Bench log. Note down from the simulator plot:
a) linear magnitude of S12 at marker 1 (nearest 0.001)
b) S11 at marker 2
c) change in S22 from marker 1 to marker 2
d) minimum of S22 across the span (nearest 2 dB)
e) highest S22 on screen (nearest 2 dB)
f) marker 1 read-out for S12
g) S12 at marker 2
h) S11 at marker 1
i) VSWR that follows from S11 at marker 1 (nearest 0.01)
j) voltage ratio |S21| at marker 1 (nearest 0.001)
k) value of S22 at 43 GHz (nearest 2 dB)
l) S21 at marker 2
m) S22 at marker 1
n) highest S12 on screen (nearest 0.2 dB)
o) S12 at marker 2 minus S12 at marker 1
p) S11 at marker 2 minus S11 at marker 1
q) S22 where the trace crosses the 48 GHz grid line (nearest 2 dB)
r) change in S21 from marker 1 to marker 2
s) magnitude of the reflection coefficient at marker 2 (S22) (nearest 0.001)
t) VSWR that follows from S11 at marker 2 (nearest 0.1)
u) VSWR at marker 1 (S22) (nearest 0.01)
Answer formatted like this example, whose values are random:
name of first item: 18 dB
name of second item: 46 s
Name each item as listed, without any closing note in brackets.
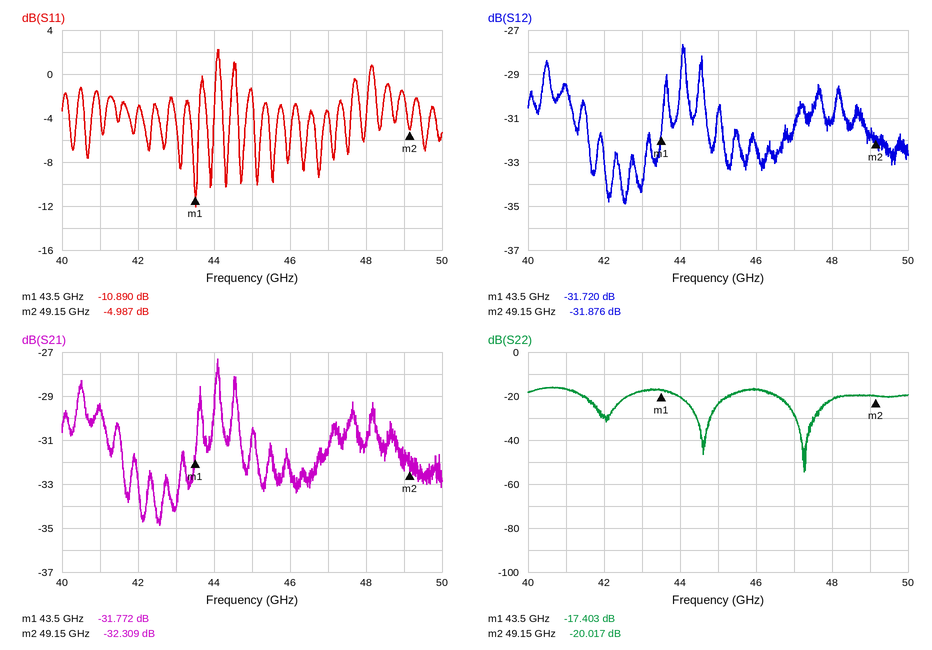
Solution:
linear magnitude of S12 at marker 1: 0.026
S11 at marker 2: -4.987 dB
change in S22 from marker 1 to marker 2: -2.614 dB
minimum of S22 across the span: -54 dB
highest S22 on screen: -16 dB
marker 1 read-out for S12: -31.720 dB
S12 at marker 2: -31.876 dB
S11 at marker 1: -10.890 dB
VSWR that follows from S11 at marker 1: 1.80
voltage ratio |S21| at marker 1: 0.026
value of S22 at 43 GHz: -18 dB
S21 at marker 2: -32.309 dB
S22 at marker 1: -17.403 dB
highest S12 on screen: -27.6 dB
S12 at marker 2 minus S12 at marker 1: -0.156 dB
S11 at marker 2 minus S11 at marker 1: 5.903 dB
S22 where the trace crosses the 48 GHz grid line: -22 dB
change in S21 from marker 1 to marker 2: -0.537 dB
magnitude of the reflection coefficient at marker 2 (S22): 0.100
VSWR that follows from S11 at marker 2: 3.6
VSWR at marker 1 (S22): 1.31
